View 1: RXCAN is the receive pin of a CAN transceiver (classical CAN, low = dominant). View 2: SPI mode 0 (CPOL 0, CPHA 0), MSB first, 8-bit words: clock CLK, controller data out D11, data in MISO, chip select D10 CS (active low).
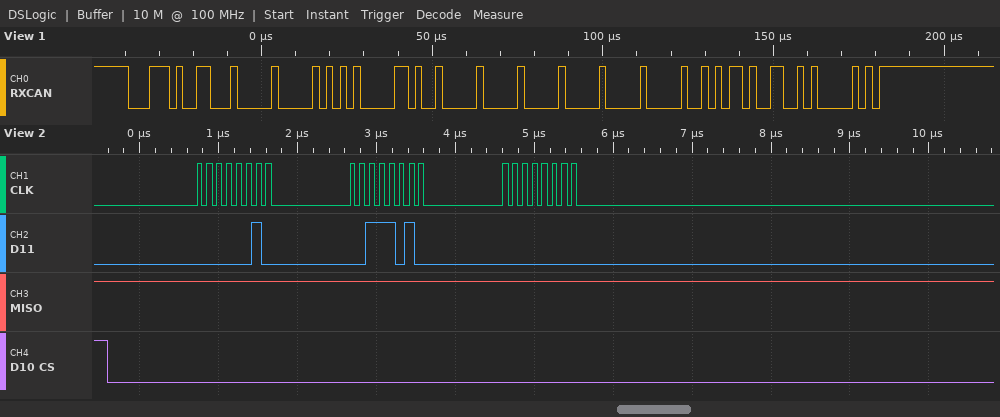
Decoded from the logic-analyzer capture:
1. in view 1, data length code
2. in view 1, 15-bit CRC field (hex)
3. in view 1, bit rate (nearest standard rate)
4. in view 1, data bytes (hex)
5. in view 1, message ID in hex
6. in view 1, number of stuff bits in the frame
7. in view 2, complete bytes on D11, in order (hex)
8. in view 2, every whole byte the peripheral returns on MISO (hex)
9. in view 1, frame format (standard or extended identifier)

8
0x1940
500 kbit/s
00 A8 29 00 00 00 00 AD
0x1D3
10
02 3A 00
FF FF FF
standard
